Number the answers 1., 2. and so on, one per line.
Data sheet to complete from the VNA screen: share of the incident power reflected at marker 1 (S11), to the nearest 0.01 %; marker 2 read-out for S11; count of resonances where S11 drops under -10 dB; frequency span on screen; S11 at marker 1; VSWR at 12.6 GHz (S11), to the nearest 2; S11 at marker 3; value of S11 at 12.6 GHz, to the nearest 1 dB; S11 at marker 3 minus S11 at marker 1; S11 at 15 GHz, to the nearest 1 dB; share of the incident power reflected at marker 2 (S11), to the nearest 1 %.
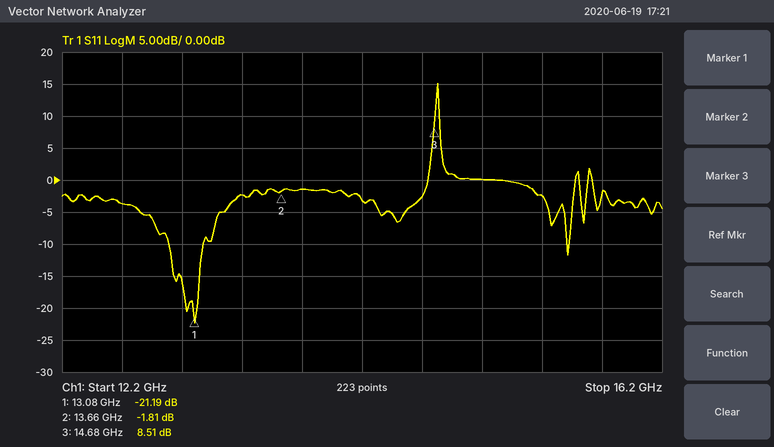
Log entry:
1. 0.76 %
2. -1.81 dB
3. 2
4. 4 GHz
5. -21.19 dB
6. 4
7. 8.51 dB
8. -4 dB
9. 29.70 dB
10. 0 dB
11. 66 %
